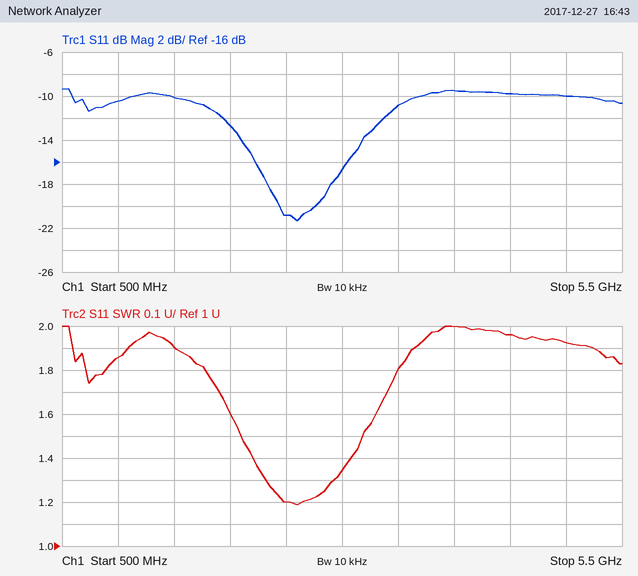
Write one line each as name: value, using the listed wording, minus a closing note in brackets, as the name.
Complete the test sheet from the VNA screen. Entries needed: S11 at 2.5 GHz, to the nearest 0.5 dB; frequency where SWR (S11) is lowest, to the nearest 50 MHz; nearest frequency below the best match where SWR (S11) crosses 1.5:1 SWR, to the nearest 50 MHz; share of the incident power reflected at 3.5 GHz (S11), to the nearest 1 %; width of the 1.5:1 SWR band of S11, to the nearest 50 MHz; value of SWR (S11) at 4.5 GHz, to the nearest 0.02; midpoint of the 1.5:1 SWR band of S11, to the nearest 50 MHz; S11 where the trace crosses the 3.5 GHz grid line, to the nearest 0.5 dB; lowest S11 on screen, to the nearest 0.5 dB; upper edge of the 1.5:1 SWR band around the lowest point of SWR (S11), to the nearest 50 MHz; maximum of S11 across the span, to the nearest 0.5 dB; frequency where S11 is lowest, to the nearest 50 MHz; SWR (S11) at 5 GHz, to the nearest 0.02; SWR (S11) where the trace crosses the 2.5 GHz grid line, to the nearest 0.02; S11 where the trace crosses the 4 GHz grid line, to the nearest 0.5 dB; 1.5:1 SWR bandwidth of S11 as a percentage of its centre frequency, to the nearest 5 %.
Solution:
S11 at 2.5 GHz, to the nearest 0.5 dB: -21.0 dB
frequency where SWR (S11) is lowest, to the nearest 50 MHz: 2.60 GHz
nearest frequency below the best match where SWR (S11) crosses 1.5:1 SWR, to the nearest 50 MHz: 2.10 GHz
share of the incident power reflected at 3.5 GHz (S11), to the nearest 1 %: 8 %
width of the 1.5:1 SWR band of S11, to the nearest 50 MHz: 1.10 GHz
value of SWR (S11) at 4.5 GHz, to the nearest 0.02: 1.96
midpoint of the 1.5:1 SWR band of S11, to the nearest 50 MHz: 2.65 GHz
S11 where the trace crosses the 3.5 GHz grid line, to the nearest 0.5 dB: -11.0 dB
lowest S11 on screen, to the nearest 0.5 dB: -21.5 dB
upper edge of the 1.5:1 SWR band around the lowest point of SWR (S11), to the nearest 50 MHz: 3.20 GHz
maximum of S11 across the span, to the nearest 0.5 dB: -9.5 dB
frequency where S11 is lowest, to the nearest 50 MHz: 2.60 GHz
SWR (S11) at 5 GHz, to the nearest 0.02: 1.92
SWR (S11) where the trace crosses the 2.5 GHz grid line, to the nearest 0.02: 1.20
S11 where the trace crosses the 4 GHz grid line, to the nearest 0.5 dB: -9.5 dB
1.5:1 SWR bandwidth of S11 as a percentage of its centre frequency, to the nearest 5 %: 40 %
